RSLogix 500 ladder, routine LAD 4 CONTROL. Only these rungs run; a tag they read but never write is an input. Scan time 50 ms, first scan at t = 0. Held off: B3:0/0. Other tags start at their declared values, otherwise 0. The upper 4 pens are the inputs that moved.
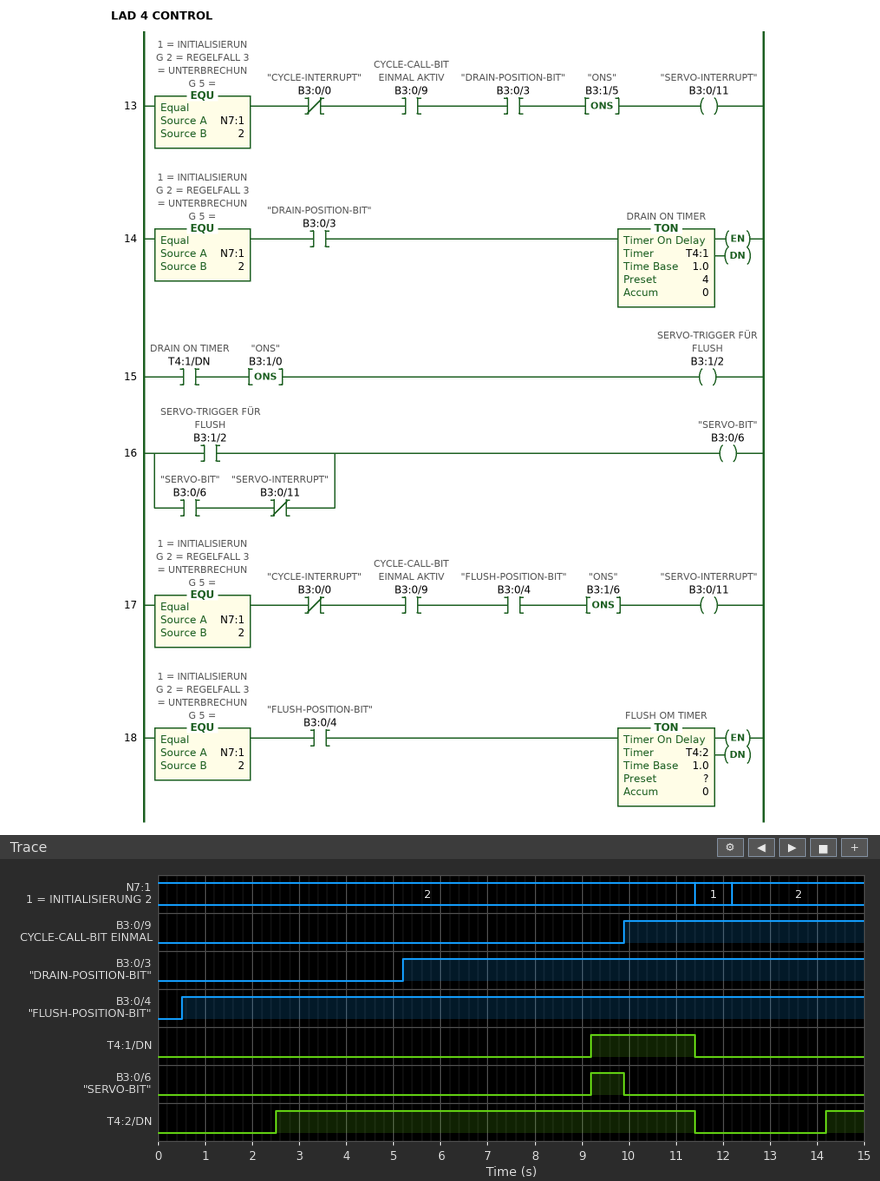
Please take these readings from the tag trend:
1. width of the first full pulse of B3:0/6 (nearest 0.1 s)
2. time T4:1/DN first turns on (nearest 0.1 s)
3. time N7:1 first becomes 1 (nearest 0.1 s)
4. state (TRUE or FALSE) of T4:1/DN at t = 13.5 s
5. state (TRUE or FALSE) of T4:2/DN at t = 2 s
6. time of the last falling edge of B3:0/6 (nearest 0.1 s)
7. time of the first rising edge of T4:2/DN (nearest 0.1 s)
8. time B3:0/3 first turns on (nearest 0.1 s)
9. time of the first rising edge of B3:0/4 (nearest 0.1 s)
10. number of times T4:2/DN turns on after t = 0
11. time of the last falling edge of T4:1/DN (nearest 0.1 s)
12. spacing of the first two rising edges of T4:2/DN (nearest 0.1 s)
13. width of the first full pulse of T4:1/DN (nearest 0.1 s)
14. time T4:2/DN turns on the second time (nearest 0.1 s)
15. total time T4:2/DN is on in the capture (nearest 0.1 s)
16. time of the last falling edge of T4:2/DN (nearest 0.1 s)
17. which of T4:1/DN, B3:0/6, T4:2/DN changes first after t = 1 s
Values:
0.7 s
9.2 s
11.4 s
FALSE
FALSE
9.9 s
2.5 s
5.2 s
0.5 s
2
11.4 s
11.7 s
2.2 s
14.2 s
9.7 s
11.4 s
T4:2/DN
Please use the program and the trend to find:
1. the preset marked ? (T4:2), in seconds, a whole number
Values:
2 s
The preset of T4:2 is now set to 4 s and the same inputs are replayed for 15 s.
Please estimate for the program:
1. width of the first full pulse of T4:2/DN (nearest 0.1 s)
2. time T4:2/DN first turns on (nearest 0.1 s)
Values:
6.9 s
4.5 s
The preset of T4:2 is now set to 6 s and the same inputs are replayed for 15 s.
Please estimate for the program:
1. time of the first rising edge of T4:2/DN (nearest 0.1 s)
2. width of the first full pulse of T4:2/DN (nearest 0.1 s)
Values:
6.5 s
4.9 s
